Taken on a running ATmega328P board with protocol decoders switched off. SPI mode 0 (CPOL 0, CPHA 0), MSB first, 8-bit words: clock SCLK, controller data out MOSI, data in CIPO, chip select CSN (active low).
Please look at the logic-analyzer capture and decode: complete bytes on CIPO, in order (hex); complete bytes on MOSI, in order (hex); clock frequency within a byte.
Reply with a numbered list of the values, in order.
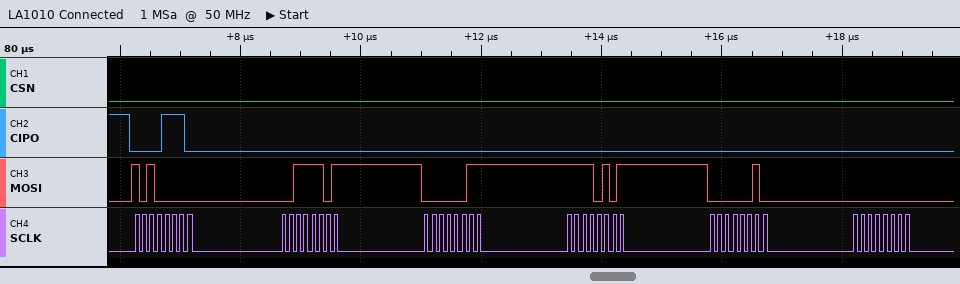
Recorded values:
1. 0E 00 00 00 00 00
2. A0 3D 03 F5 02 00
3. 8 MHz
